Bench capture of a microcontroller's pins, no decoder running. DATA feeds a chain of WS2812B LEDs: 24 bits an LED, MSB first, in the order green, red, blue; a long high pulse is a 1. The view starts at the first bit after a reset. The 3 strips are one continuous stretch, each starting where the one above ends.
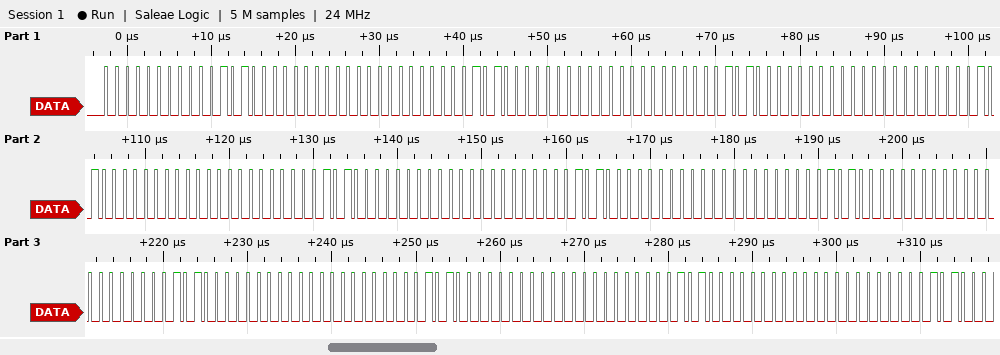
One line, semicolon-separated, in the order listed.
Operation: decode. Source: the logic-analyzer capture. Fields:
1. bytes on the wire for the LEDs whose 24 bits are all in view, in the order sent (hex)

00 14 00 00 14 00 00 14 00 00 14 00 00 14 00 00 14 00 00 14 00 00 14 00 00 14 00 00 14 00
